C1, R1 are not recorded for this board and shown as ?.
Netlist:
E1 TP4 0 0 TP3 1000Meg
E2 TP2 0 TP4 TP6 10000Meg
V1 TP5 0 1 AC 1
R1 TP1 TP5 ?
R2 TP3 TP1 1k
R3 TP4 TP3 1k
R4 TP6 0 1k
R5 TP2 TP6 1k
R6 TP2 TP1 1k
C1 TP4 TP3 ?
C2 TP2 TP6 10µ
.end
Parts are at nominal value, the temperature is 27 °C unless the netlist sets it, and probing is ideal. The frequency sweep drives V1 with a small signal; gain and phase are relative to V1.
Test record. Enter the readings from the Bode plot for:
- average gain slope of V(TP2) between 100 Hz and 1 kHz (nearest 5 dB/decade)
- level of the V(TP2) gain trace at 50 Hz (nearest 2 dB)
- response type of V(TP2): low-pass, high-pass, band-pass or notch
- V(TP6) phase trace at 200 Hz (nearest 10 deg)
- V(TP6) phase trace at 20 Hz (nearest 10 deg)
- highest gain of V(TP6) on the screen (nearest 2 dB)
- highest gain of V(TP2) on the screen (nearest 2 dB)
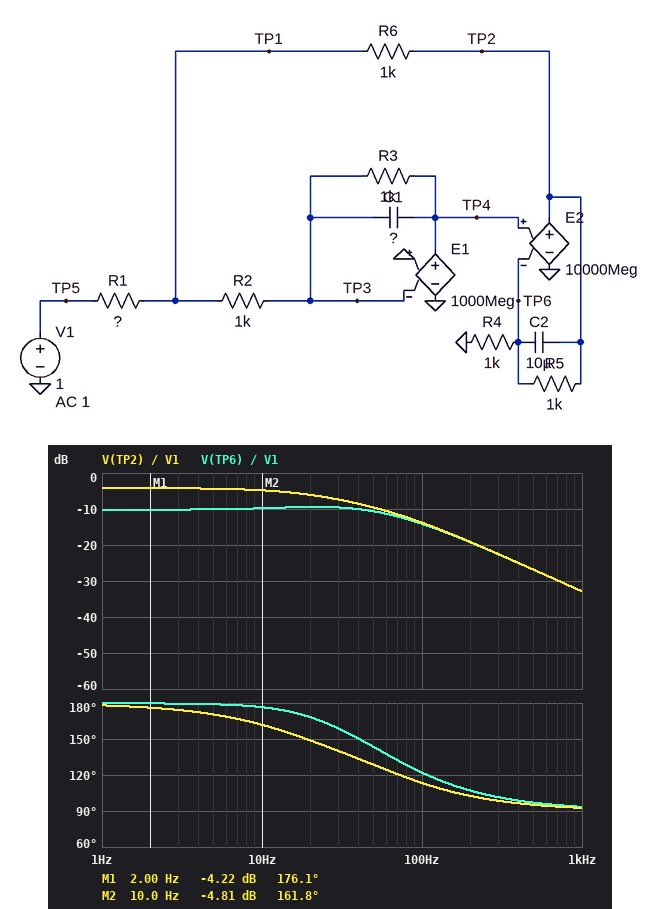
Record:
-20 dB/decade
-10 dB
low-pass
110 deg
170 deg
-10 dB
-4 dB
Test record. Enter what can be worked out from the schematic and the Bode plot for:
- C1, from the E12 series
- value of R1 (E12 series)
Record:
3.3 µF
560 Ω
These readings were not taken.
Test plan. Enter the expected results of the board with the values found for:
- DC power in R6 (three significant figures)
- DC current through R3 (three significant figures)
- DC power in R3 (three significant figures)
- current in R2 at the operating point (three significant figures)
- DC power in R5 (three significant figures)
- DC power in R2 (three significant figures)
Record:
857 µW
309 µA
95.3 µW
309 µA
95.3 µW
95.3 µW
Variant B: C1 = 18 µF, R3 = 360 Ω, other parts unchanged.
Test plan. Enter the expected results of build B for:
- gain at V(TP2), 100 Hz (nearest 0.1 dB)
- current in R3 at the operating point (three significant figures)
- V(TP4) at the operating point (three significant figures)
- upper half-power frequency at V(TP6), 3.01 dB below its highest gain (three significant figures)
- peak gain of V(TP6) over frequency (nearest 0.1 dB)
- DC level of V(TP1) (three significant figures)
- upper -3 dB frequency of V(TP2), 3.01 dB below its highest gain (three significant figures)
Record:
-27.6 dB
396 µA
-143 mV
31.9 Hz
-16.9 dB
396 mV
16.9 Hz
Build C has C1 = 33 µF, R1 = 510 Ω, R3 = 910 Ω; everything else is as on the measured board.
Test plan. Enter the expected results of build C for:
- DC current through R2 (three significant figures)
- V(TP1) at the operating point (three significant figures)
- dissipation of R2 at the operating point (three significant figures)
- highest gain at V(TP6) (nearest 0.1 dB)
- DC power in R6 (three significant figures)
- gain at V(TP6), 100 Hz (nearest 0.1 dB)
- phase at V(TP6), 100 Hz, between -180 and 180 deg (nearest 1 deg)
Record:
339 µA
339 mV
115 µW
-10.2 dB
915 µW
-32.4 dB
94 deg
